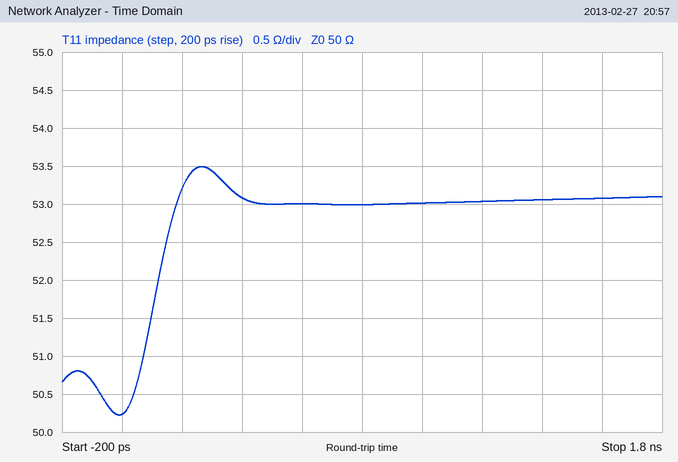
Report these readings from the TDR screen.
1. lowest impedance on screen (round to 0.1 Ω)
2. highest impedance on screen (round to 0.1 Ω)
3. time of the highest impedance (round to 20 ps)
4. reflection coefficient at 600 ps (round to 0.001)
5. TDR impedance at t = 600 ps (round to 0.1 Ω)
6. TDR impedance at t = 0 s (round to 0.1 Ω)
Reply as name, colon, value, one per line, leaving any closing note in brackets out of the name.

lowest impedance on screen: 50.2 Ω
highest impedance on screen: 53.5 Ω
time of the highest impedance: 260 ps
reflection coefficient at 600 ps: +0.029
TDR impedance at t = 600 ps: 53.0 Ω
TDR impedance at t = 0 s: 50.2 Ω
